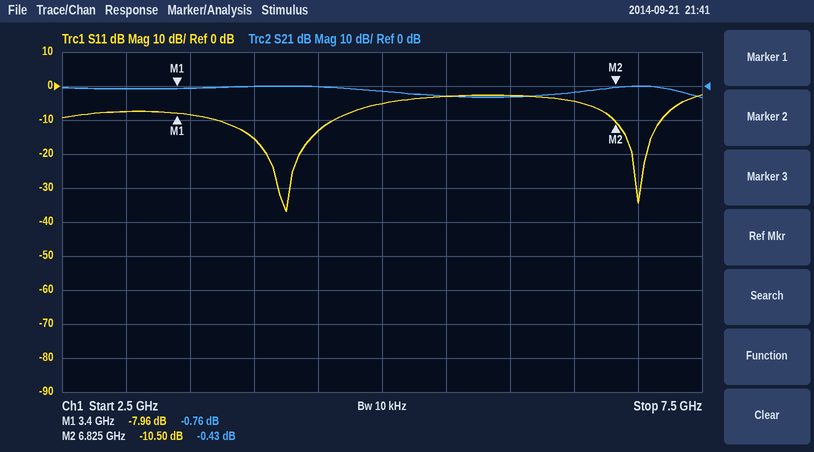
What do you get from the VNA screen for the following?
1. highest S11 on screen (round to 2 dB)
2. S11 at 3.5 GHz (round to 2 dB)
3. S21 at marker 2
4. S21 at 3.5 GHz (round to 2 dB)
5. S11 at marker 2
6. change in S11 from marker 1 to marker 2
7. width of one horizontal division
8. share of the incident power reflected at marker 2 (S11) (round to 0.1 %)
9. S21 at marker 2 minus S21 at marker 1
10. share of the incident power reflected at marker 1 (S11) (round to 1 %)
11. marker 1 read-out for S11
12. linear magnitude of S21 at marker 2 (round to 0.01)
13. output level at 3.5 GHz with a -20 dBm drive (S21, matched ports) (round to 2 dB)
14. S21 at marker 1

-2 dB
-8 dB
-0.43 dB
0 dB
-10.50 dB
-2.54 dB
500 MHz
8.9 %
0.33 dB
16 %
-7.96 dB
0.95
-20 dBm
-0.76 dB
